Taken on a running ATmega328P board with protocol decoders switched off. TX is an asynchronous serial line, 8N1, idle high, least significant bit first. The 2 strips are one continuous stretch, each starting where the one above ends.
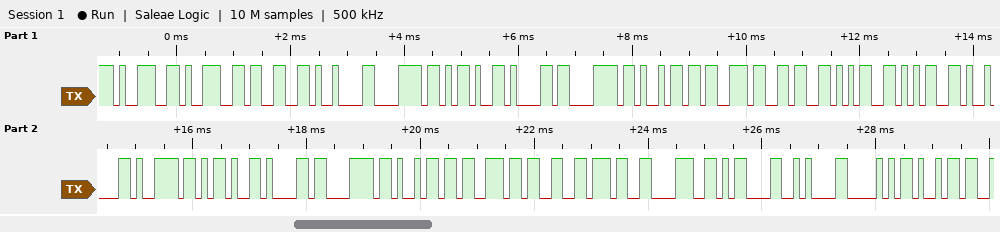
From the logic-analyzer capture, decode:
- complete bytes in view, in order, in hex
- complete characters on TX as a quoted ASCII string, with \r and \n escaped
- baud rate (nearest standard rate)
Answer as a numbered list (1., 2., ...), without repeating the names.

1. 39 39 33 09 78 2D 61 78 69 73 36 35 35 09 79 2D 61 78 69 73 33 37 38 0D 0A 50 69
2. "993\tx-axis655\ty-axis378\r\nPi"
3. 9600 baud
